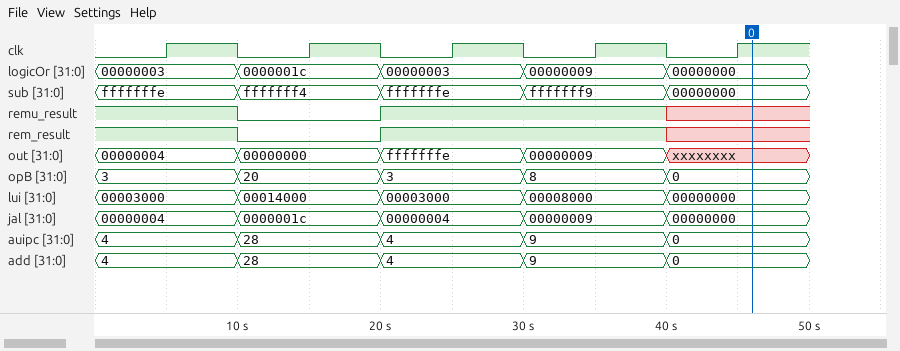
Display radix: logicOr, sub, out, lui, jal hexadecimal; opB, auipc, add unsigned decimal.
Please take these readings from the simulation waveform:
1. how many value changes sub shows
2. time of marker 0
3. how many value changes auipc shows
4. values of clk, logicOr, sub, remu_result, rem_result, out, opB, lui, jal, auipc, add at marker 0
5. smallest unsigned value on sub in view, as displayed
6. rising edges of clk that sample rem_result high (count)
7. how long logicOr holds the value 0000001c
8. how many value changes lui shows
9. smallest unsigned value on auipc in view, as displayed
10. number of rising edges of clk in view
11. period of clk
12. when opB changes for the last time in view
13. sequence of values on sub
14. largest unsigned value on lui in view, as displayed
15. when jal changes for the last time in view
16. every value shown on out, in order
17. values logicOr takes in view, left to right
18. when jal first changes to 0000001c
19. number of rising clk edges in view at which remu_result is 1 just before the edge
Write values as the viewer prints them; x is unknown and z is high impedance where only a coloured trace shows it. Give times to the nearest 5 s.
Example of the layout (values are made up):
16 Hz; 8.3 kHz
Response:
4; 45 s; 4; clk=1, logicOr=00000000, sub=00000000, remu_result=x, rem_result=x, out=xxxxxxxx, opB=0, lui=00000000, jal=00000000, auipc=0, add=0; 00000000; 3; 10 s; 4; 0; 5; 10 s; 40 s; fffffffe, fffffff4, fffffffe, fffffff9, 00000000; 00014000; 40 s; 00000004, 00000000, fffffffe, 00000009, xxxxxxxx; 00000003, 0000001c, 00000003, 00000009, 00000000; 10 s; 3
